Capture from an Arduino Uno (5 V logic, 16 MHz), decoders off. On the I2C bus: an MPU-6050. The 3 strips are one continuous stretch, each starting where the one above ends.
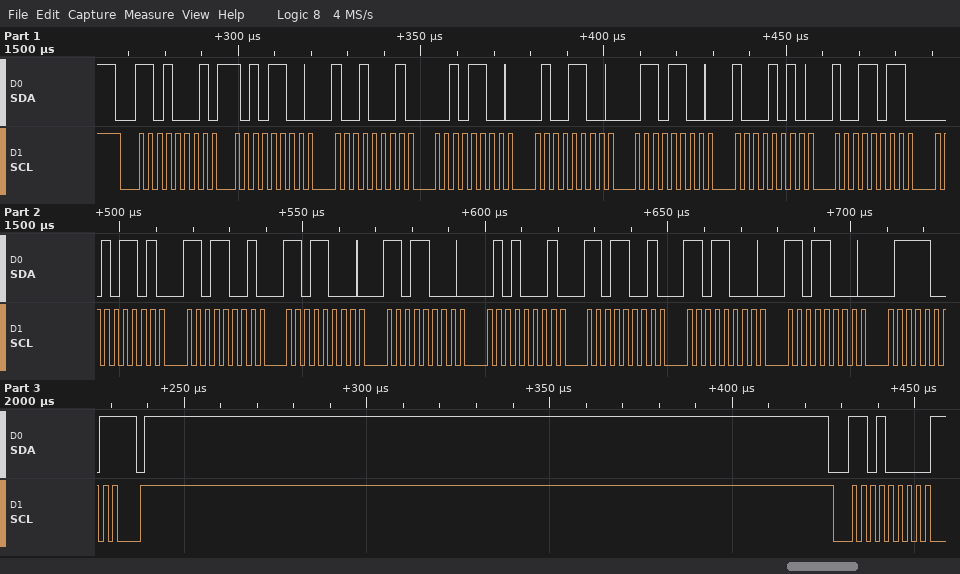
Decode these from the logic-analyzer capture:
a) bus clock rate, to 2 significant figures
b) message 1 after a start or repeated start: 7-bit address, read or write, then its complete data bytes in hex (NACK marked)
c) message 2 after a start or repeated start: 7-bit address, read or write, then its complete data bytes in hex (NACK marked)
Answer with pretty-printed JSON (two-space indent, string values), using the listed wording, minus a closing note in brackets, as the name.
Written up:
{
  "bus clock rate, to 2 significant figures": "400 kHz",
  "message 1 after a start or repeated start: 7-bit address, read or write, then its complete data bytes in hex": "0x68 read: AC 91 2C 4C 6C 8A 9B 2D D9 D8 D8 51 D9 D8 D8 79 NACK",
  "message 2 after a start or repeated start: 7-bit address, read or write, then its complete data bytes in hex": "0x68 write"
}
